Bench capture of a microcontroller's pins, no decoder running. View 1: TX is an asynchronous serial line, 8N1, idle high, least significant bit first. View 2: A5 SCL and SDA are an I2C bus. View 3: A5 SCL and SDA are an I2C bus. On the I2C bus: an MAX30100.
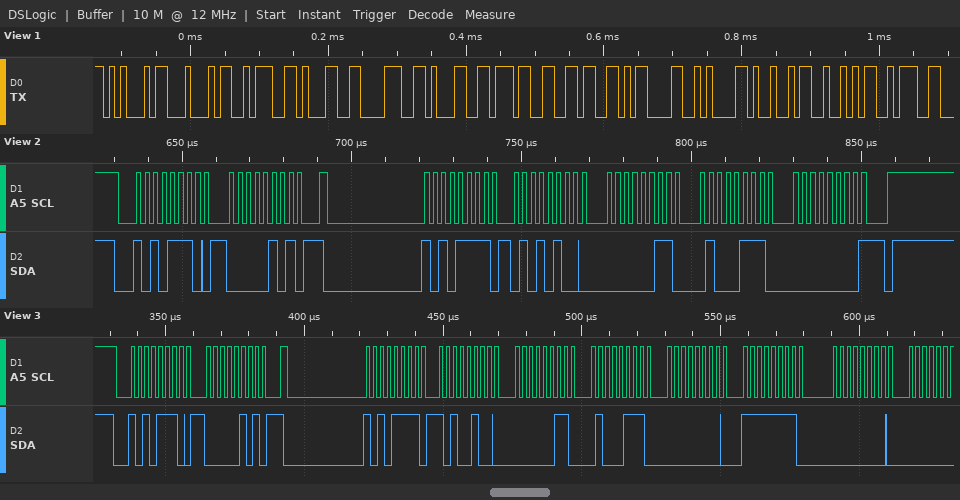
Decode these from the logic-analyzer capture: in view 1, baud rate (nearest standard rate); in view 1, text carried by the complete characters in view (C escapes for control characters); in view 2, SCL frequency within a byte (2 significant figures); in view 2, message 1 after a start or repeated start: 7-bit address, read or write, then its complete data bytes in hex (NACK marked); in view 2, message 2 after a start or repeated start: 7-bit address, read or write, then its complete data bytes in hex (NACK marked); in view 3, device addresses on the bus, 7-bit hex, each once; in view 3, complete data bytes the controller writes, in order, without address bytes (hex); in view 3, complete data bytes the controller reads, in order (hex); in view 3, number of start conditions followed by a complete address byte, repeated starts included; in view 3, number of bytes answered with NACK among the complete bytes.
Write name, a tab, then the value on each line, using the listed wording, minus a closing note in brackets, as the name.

in view 1, baud rate	115200 baud
in view 1, text carried by the complete characters in view	"ED:18176\r\nIR:"
in view 2, SCL frequency within a byte	400 kHz
in view 2, message 1 after a start or repeated start: 7-bit address, read or write, then its complete data bytes in hex	0x57 write: 05
in view 2, message 2 after a start or repeated start: 7-bit address, read or write, then its complete data bytes in hex	0x57 read: 54 03 47 00 NACK
in view 3, device addresses on the bus, 7-bit hex, each once	0x57
in view 3, complete data bytes the controller writes, in order, without address bytes	05
in view 3, complete data bytes the controller reads, in order	A4 03 47 00 FF 00
in view 3, number of start conditions followed by a complete address byte, repeated starts included	2
in view 3, number of bytes answered with NACK among the complete bytes	0
